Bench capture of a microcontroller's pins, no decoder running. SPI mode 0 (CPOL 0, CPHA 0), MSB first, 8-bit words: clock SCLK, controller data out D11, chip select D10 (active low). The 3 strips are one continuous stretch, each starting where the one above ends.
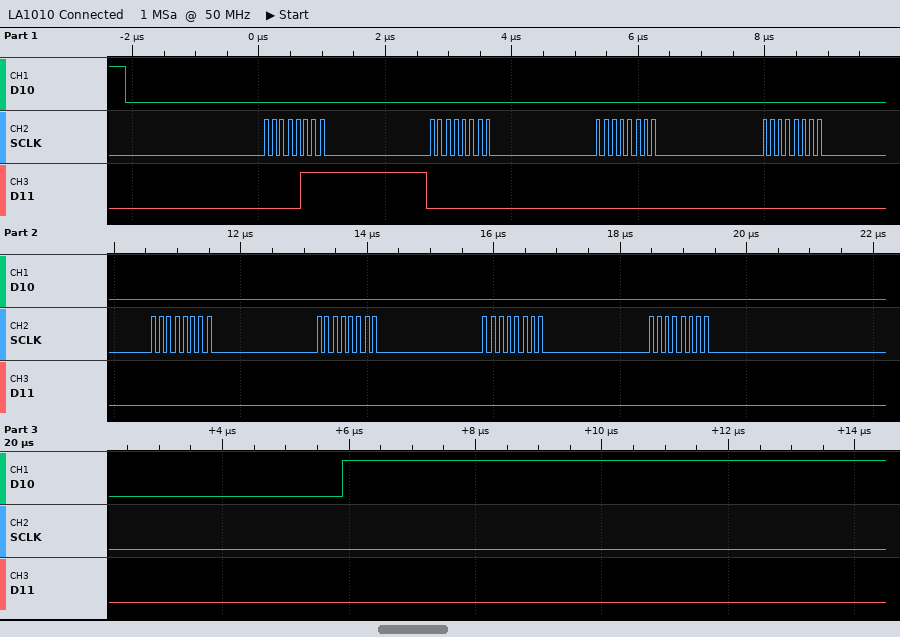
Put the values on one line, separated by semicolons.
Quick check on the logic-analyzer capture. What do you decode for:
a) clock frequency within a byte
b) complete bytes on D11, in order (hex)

8 MHz; 0x07 0x00 0x00 0x00 0x00 0x00 0x00 0x00
